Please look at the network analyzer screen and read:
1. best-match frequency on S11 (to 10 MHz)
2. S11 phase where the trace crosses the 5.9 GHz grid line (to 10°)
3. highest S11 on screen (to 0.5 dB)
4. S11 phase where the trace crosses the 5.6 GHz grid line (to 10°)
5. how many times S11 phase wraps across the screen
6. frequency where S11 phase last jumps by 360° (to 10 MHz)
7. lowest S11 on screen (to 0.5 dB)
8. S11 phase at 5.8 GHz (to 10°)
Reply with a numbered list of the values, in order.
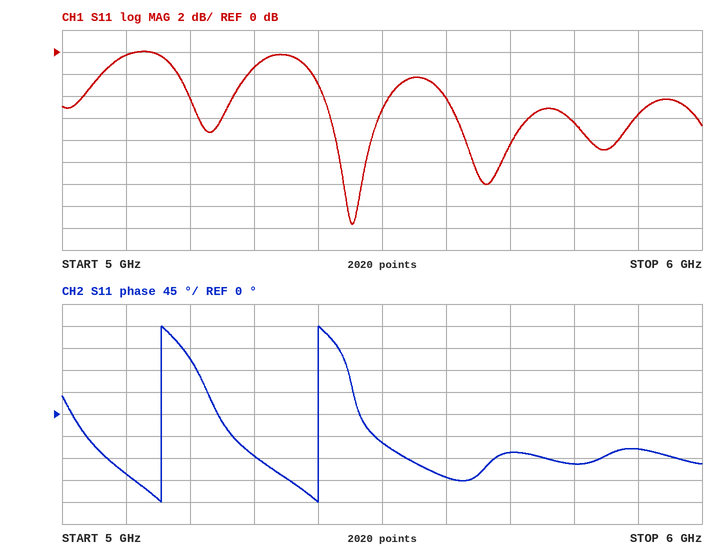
1. 5.45 GHz
2. -70°
3. 0.0 dB
4. -130°
5. 2
6. 5.40 GHz
7. -15.5 dB
8. -100°
